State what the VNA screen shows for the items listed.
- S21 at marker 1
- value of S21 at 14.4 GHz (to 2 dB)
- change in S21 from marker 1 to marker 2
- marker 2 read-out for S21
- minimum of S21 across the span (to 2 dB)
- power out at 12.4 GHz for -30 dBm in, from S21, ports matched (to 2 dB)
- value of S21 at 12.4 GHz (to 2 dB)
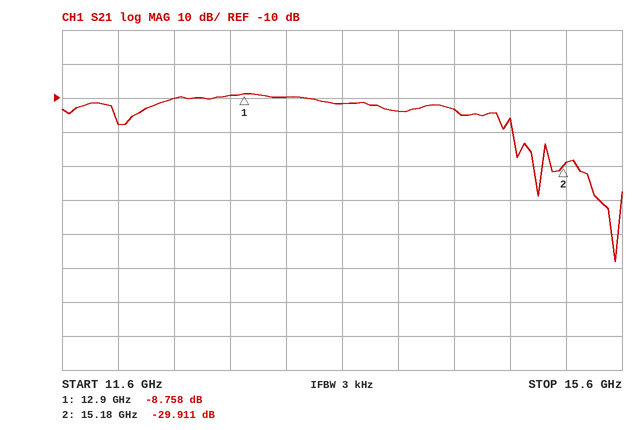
-8.758 dB
-14 dB
-21.153 dB
-29.911 dB
-58 dB
-40 dBm
-10 dB
